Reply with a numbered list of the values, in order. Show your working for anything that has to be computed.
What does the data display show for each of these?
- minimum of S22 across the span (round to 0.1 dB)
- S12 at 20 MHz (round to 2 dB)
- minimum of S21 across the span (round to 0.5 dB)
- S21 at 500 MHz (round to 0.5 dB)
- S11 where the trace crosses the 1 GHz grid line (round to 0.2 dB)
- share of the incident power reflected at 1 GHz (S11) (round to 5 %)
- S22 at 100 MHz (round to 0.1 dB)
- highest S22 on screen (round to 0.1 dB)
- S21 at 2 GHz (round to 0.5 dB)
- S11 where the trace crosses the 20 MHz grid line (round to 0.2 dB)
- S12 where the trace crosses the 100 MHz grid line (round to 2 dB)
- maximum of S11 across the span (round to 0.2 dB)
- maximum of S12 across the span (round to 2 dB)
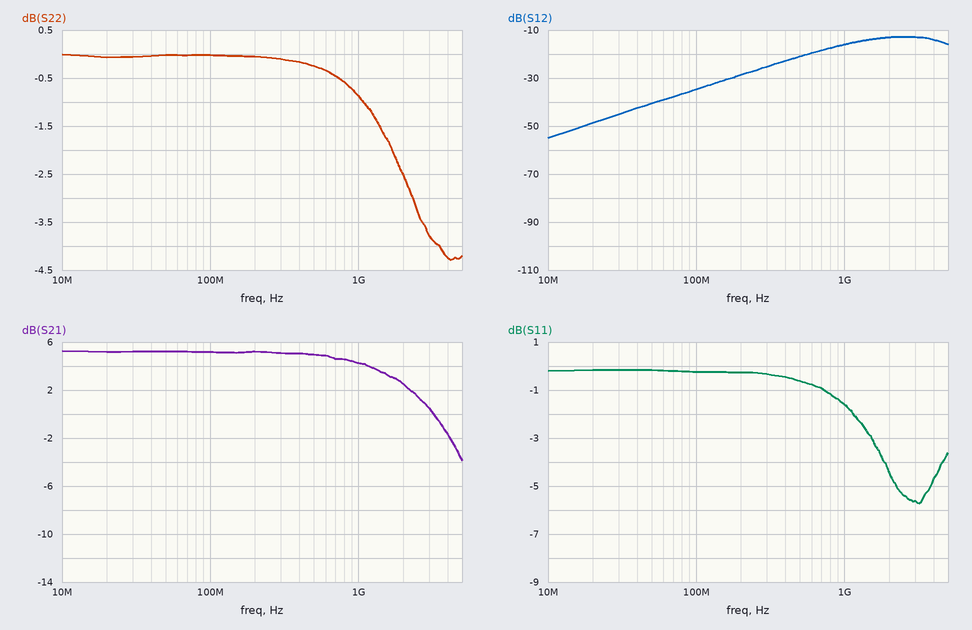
1. -4.3 dB
2. -48 dB
3. -4.0 dB
4. 5.0 dB
5. -1.6 dB
6. 10^(-1.6/10) ≈ 69.2 %, so 70 % to the nearest 5 %
7. 0.0 dB
8. 0.0 dB
9. 2.5 dB
10. -0.2 dB
11. -34 dB
12. -0.2 dB
13. -12 dB
